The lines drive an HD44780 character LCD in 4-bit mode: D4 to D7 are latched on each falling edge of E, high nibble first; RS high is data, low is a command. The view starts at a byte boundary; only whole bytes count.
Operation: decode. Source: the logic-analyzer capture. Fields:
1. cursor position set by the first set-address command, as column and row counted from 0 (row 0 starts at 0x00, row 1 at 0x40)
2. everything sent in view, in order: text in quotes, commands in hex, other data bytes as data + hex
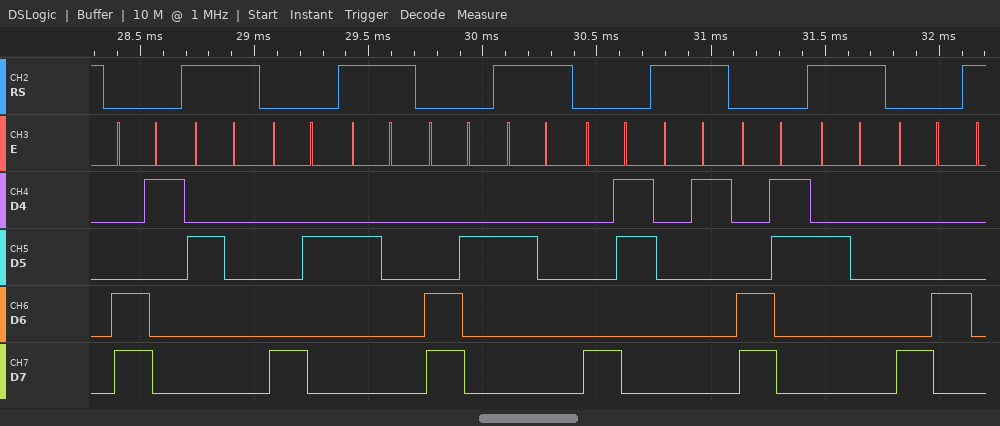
column 1, row 1
0xC1 " " 0x82 " " 0xC2 " " 0x83 data 01 0xC3 " " 0x84
